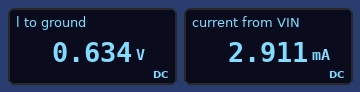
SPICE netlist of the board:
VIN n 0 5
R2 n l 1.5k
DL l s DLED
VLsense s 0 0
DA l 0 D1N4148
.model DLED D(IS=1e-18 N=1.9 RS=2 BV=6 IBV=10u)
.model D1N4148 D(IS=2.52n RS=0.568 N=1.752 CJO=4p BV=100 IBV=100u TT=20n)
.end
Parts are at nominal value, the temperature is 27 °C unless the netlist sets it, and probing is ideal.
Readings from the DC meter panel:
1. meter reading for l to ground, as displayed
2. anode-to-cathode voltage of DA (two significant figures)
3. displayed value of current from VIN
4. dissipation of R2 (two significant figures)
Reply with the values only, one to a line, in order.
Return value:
0.634 V
630 mV
2.911 mA
13 mW
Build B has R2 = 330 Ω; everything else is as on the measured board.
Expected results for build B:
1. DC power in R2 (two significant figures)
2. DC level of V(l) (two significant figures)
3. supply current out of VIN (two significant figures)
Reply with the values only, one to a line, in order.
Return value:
56 mW
710 mV
13 mA
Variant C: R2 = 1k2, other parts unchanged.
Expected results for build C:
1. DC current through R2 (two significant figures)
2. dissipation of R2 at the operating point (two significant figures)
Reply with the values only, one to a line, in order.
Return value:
3.6 mA
16 mW
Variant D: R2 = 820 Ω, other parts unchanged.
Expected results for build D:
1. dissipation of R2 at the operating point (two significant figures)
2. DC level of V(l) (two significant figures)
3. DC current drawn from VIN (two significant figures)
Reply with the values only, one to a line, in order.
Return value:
23 mW
660 mV
5.3 mA
